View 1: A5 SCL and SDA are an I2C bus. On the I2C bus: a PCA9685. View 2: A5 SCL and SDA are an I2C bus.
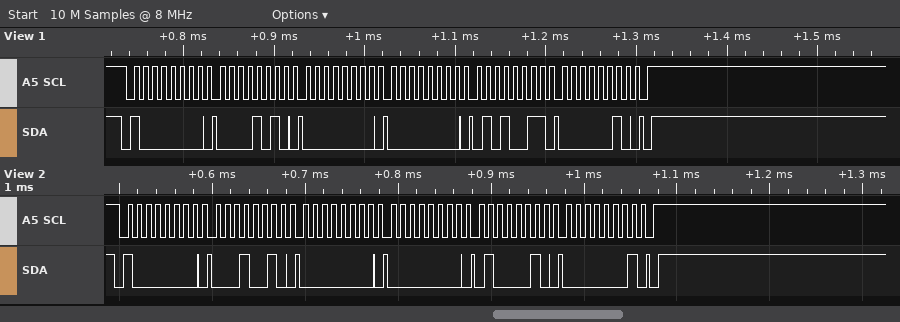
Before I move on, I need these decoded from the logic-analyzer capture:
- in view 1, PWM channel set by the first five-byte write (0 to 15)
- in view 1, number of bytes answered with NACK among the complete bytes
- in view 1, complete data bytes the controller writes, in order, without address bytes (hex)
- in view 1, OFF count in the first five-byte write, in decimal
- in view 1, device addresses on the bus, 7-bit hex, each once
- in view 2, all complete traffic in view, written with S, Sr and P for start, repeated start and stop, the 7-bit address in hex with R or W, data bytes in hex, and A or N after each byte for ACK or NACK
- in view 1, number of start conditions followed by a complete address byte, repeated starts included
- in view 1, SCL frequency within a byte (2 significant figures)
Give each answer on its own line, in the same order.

1
0
0A 00 00 53 02
595
0x40
S 40W A 12 A 00 A 00 A 42 A 01 A P
1
100 kHz
